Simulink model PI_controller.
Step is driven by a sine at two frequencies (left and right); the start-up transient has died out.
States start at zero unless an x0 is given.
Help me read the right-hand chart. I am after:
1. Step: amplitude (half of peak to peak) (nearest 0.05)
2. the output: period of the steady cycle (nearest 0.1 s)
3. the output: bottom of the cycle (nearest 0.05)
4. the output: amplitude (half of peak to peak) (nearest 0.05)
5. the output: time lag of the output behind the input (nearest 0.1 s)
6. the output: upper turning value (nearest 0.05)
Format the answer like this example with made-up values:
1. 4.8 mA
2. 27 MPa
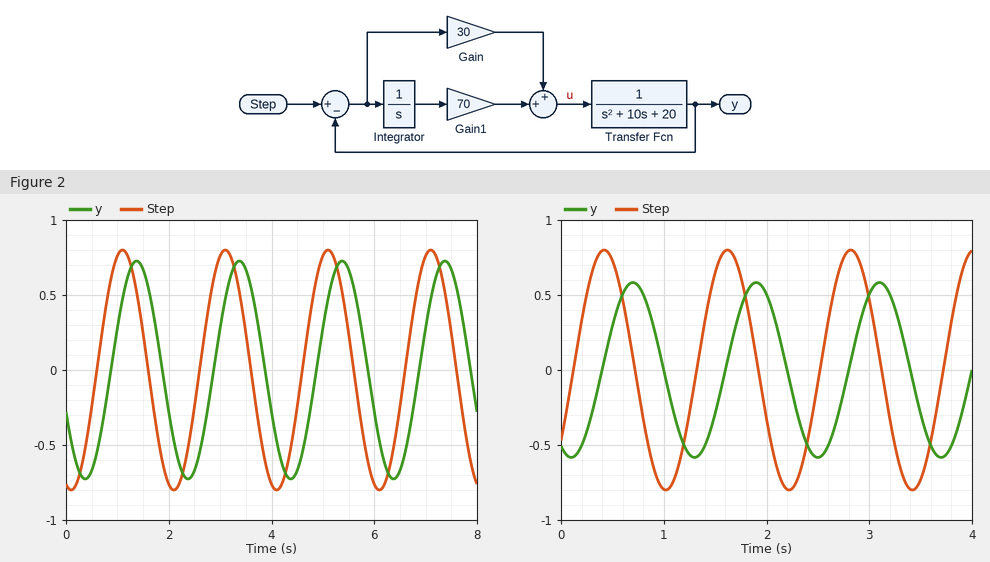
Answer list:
1. 0.80
2. 1.2 s
3. -0.60
4. 0.60
5. 0.3 s
6. 0.60
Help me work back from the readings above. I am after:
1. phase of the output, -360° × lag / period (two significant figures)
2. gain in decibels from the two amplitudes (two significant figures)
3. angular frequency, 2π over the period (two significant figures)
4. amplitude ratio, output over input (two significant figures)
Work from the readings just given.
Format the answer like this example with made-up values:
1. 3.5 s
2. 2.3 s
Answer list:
1. -90°
2. -2.5 dB
3. 5.2 rad/s
4. 0.75
